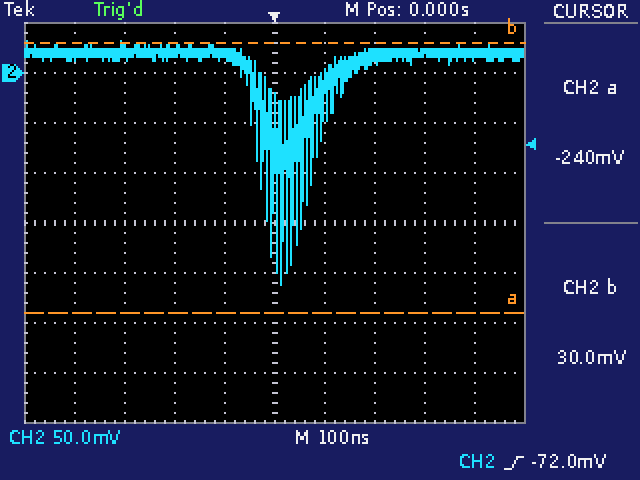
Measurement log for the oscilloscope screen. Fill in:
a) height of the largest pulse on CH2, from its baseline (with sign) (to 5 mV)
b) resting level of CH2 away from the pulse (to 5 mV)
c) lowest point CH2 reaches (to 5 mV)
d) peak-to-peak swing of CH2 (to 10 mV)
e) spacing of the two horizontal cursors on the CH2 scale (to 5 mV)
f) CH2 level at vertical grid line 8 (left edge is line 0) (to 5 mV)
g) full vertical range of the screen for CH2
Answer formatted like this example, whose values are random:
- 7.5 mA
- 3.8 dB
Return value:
- -230 mV
- 20 mV
- -210 mV
- 240 mV
- 270 mV
- 20 mV
- 400 mV
